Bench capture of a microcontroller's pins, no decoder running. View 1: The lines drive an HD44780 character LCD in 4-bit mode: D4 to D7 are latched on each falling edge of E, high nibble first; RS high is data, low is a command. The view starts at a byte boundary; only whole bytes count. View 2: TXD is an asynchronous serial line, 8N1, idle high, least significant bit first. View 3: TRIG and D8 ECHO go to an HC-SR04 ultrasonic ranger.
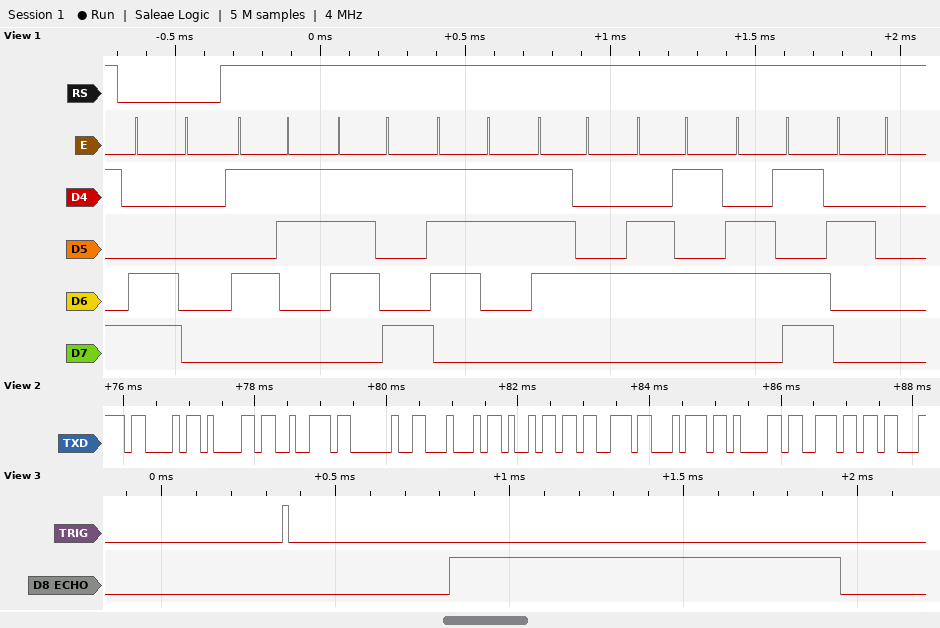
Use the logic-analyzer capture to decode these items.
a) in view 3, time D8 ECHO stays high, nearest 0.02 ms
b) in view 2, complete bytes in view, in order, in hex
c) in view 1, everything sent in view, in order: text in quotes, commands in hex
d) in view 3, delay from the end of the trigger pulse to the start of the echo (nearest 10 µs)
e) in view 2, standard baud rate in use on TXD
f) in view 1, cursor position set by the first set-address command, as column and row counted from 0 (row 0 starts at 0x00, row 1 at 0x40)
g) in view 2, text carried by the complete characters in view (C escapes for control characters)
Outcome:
1.12 ms
0x43 0x61 0x72 0x20 0x44 0x69 0x73 0x74 0x61 0x6E
0xC0 "System "
460 µs
9600 baud
column 0, row 1
"Car Distan"
